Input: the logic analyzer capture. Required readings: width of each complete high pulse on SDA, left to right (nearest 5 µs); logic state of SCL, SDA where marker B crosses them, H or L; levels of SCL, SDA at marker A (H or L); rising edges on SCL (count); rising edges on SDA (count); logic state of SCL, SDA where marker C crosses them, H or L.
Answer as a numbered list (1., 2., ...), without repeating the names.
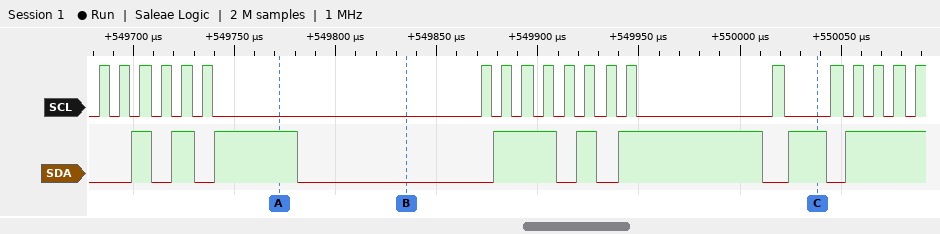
1. 10 µs, 10 µs, 40 µs, 30 µs, 10 µs, 70 µs, 20 µs
2. SCL=L, SDA=L
3. SCL=L, SDA=H
4. 20
5. 8
6. SCL=L, SDA=H
